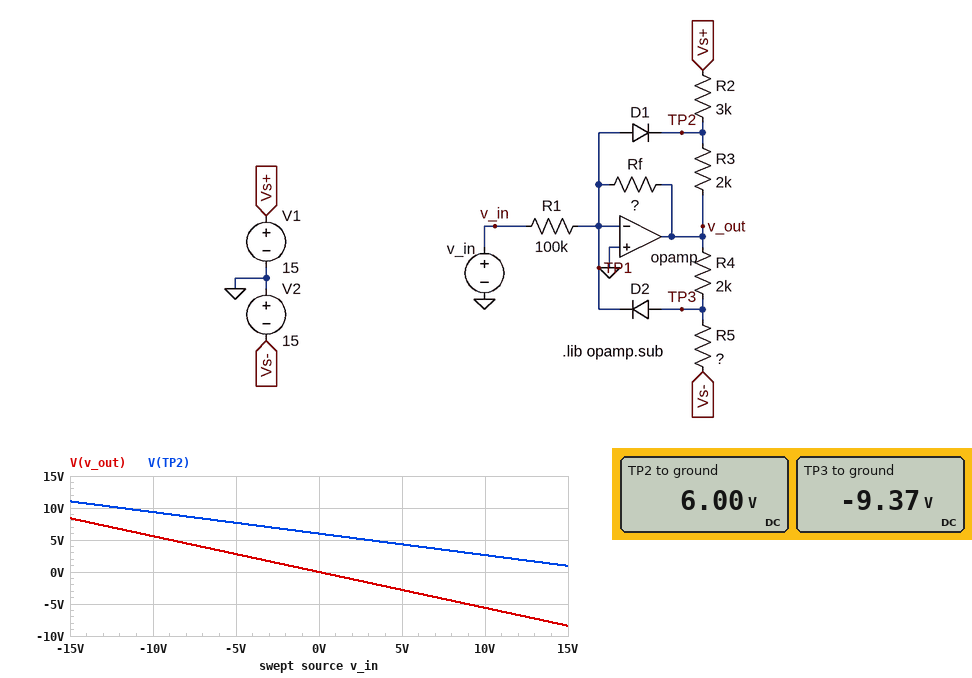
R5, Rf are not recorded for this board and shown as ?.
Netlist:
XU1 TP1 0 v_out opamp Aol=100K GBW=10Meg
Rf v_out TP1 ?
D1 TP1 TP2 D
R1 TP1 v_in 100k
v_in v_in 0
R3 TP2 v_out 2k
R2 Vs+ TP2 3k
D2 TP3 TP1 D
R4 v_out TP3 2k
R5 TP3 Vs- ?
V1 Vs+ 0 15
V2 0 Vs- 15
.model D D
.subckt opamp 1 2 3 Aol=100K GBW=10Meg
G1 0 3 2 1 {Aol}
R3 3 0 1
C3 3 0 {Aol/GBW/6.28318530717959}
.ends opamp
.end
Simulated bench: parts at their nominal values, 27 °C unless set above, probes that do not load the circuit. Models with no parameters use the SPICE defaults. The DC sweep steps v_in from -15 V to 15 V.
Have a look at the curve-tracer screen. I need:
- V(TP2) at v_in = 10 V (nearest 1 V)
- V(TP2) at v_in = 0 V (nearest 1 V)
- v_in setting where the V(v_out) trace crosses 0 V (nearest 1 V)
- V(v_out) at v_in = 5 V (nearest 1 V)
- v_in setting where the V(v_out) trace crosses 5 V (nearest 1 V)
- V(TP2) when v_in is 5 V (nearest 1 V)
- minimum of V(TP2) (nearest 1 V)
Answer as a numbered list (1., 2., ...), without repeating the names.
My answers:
1. 3 V
2. 6 V
3. 0 V
4. -3 V
5. -9 V
6. 4 V
7. 1 V
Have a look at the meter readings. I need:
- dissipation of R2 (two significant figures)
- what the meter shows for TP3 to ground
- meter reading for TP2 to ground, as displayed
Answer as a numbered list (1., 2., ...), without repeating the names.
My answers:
1. 27 mW
2. -9.37 V
3. 6.00 V
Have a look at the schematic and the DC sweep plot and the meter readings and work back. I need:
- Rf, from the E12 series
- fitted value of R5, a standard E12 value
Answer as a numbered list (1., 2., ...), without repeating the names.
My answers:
1. 56 kΩ
2. 1.2 kΩ
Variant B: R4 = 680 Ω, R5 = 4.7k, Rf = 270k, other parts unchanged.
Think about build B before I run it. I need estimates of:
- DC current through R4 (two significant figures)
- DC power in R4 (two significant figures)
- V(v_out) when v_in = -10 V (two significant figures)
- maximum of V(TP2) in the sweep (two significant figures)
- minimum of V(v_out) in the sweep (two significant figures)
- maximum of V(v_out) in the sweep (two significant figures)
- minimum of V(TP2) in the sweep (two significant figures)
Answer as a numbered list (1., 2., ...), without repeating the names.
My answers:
1. 2.8 mA
2. 5.3 mW
3. 2.9 V
4. 7.8 V
5. -11 V
6. 3.0 V
7. -600 mV
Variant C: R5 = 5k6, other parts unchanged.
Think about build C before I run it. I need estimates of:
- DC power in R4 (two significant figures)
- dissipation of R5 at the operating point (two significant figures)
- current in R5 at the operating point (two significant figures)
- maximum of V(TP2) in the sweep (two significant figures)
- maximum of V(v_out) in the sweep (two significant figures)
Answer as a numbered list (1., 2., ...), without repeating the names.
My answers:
1. 7.8 mW
2. 22 mW
3. 2.0 mA
4. 9.7 V
5. 6.2 V
